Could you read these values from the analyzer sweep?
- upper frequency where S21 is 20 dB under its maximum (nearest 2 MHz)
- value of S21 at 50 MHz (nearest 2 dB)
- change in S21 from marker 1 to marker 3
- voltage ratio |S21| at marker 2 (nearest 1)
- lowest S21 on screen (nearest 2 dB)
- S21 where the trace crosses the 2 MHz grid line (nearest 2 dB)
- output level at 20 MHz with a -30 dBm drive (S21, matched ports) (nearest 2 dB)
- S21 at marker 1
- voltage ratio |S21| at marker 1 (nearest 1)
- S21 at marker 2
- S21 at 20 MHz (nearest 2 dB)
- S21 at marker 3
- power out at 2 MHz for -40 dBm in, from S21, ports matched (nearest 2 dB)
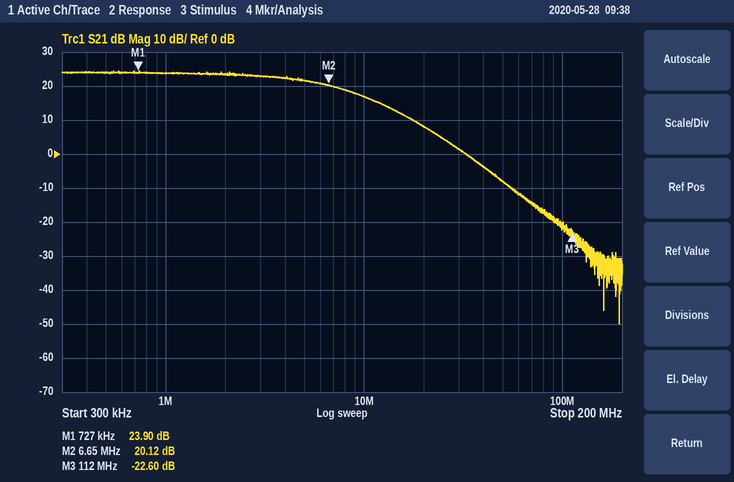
24 MHz
-8 dB
-46.50 dB
10
-50 dB
24 dB
-22 dBm
23.90 dB
16
20.12 dB
8 dB
-22.60 dB
-16 dBm
